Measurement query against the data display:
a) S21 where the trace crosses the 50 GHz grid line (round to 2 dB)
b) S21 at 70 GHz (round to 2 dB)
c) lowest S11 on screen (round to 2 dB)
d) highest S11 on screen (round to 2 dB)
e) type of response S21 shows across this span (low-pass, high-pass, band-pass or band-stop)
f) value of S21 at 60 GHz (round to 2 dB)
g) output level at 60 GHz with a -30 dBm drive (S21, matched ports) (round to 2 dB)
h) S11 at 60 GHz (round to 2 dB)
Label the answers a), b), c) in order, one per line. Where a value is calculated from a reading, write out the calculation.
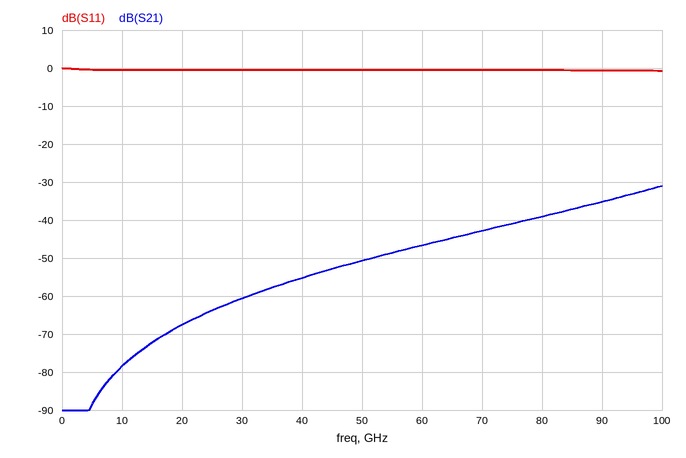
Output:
a) -50 dB
b) -42 dB
c) 0 dB
d) 0 dB
e) high-pass
f) -46 dB
g) -30 dBm + (-46 dB) = -76 dBm
h) 0 dB
